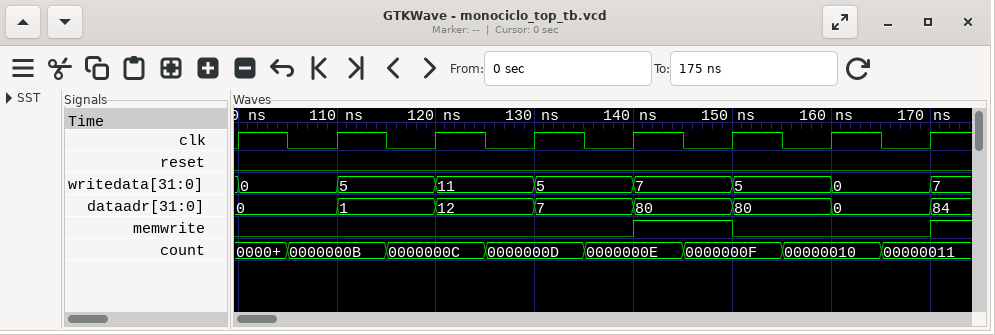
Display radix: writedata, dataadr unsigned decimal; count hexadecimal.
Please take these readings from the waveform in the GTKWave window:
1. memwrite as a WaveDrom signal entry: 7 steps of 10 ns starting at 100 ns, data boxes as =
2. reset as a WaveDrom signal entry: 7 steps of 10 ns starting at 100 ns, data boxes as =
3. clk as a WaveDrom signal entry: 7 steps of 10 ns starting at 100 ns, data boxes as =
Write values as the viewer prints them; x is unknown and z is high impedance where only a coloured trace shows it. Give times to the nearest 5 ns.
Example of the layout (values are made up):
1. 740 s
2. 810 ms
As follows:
1. {name: 'memwrite', wave: '0...10.'}
2. {name: 'reset', wave: '0......'}
3. {name: 'clk', wave: 'p......'}
